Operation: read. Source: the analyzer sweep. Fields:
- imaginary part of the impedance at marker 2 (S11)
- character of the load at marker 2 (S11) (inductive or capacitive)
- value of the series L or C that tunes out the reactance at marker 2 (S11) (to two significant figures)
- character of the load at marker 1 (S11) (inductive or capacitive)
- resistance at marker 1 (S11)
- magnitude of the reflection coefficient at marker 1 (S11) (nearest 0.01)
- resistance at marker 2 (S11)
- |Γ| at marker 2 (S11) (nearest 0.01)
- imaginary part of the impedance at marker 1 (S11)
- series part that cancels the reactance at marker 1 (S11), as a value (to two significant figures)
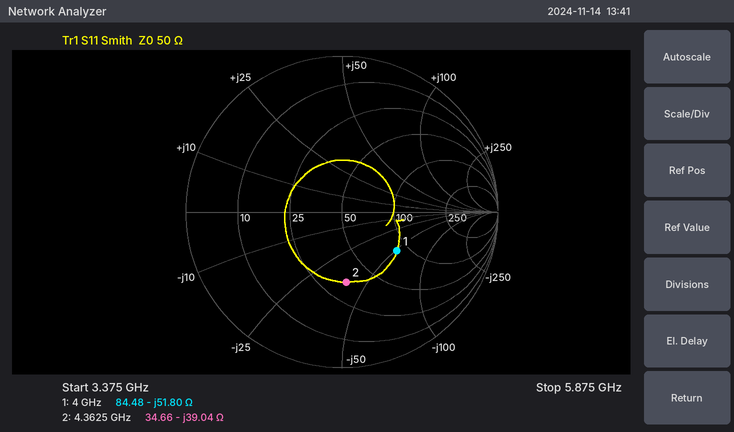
-39.04 Ω
capacitive
1.4 nH
capacitive
84.48 Ω
0.43
34.66 Ω
0.45
-51.80 Ω
2.1 nH
